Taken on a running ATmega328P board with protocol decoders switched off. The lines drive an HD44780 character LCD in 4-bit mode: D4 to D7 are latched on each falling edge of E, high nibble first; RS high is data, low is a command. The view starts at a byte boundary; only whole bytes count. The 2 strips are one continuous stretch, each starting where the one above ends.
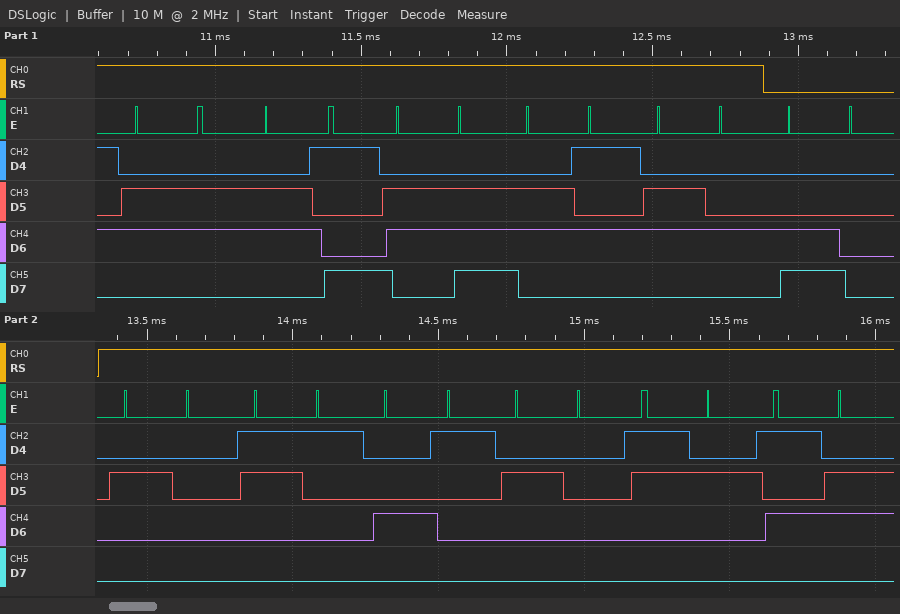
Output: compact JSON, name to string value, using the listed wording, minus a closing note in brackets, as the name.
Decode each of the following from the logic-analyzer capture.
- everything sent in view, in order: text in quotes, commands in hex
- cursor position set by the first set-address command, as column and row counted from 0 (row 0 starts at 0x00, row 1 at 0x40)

{"everything sent in view, in order: text in quotes, commands in hex": "\"fined\" 0xC0 \" 1A 2V\"", "cursor position set by the first set-address command, as column and row counted from 0": "column 0, row 1"}
